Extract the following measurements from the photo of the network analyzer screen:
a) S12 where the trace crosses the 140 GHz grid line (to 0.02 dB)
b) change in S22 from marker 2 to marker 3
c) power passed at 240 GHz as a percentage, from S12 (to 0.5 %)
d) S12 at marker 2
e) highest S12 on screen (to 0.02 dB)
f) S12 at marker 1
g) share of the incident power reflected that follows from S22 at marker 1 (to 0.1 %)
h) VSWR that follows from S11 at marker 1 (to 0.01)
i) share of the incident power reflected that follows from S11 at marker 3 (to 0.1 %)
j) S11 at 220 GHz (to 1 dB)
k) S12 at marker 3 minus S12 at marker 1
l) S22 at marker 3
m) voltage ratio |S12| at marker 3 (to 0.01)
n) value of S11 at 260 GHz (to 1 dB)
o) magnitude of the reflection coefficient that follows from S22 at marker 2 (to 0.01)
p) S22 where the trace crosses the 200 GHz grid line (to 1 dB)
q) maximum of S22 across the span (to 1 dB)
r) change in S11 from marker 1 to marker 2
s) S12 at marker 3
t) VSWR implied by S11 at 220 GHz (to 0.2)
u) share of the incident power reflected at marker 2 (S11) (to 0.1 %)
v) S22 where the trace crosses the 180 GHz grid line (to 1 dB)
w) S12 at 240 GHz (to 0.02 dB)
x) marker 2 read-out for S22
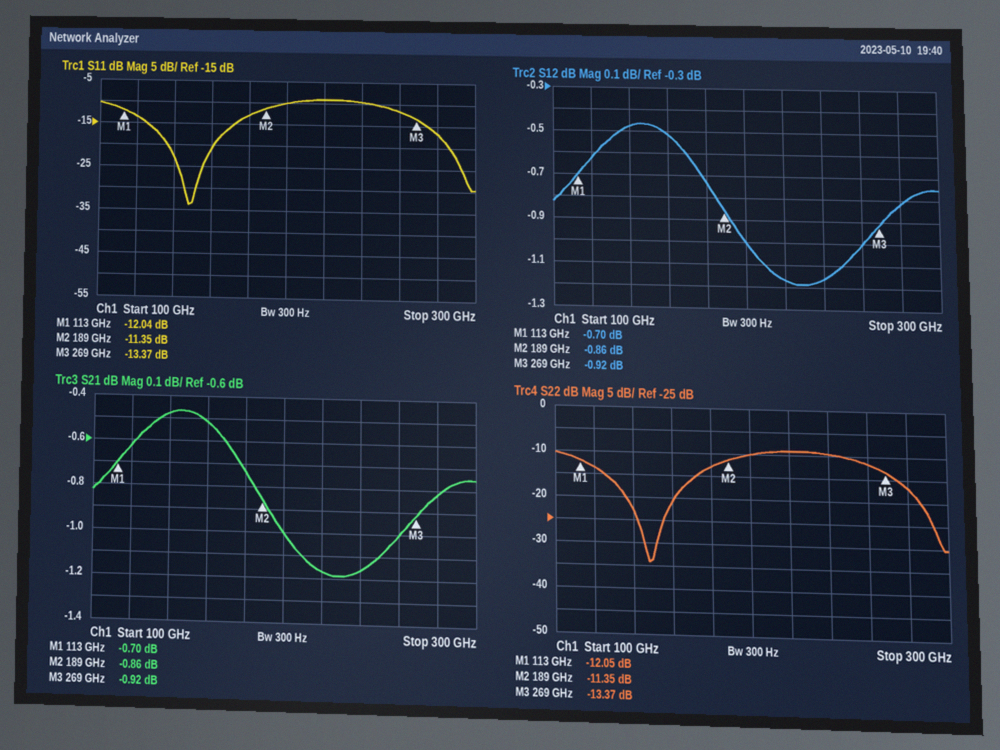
-0.48 dB
-2.02 dB
76.5 %
-0.86 dB
-0.46 dB
-0.70 dB
6.2 %
1.67
4.6 %
-9 dB
-0.22 dB
-13.37 dB
0.90
-12 dB
0.27
-10 dB
-9 dB
0.69 dB
-0.92 dB
2.0
7.3 %
-13 dB
-1.16 dB
-11.35 dB
